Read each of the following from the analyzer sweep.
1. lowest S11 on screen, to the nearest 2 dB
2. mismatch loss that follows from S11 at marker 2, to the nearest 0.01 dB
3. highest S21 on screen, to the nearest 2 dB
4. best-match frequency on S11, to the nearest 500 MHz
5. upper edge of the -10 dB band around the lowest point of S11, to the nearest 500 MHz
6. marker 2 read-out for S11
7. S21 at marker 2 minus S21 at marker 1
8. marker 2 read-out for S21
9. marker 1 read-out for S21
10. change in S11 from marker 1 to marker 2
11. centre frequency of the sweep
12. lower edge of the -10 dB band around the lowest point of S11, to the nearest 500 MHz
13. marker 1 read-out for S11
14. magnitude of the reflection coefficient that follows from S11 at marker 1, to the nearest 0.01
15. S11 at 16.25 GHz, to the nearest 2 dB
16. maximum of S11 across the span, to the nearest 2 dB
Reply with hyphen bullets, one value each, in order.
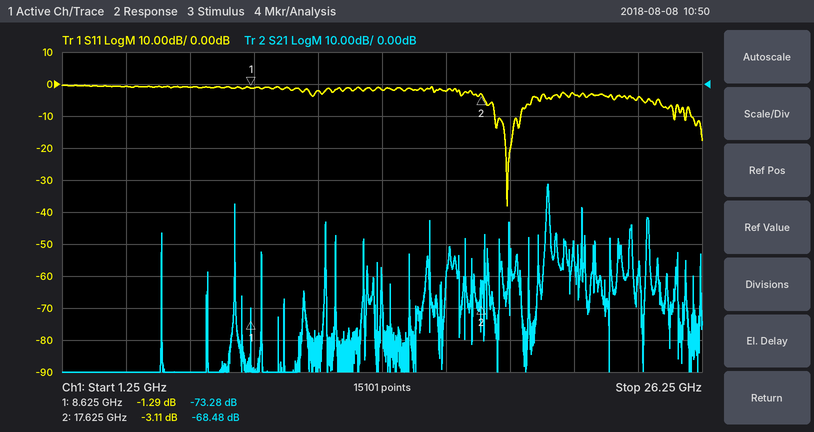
- -38 dB
- 2.91 dB
- -32 dB
- 18.5 GHz
- 19.0 GHz
- -3.11 dB
- 4.80 dB
- -68.48 dB
- -73.28 dB
- -1.82 dB
- 13.75 GHz
- 18.0 GHz
- -1.29 dB
- 0.86
- -2 dB
- 0 dB
